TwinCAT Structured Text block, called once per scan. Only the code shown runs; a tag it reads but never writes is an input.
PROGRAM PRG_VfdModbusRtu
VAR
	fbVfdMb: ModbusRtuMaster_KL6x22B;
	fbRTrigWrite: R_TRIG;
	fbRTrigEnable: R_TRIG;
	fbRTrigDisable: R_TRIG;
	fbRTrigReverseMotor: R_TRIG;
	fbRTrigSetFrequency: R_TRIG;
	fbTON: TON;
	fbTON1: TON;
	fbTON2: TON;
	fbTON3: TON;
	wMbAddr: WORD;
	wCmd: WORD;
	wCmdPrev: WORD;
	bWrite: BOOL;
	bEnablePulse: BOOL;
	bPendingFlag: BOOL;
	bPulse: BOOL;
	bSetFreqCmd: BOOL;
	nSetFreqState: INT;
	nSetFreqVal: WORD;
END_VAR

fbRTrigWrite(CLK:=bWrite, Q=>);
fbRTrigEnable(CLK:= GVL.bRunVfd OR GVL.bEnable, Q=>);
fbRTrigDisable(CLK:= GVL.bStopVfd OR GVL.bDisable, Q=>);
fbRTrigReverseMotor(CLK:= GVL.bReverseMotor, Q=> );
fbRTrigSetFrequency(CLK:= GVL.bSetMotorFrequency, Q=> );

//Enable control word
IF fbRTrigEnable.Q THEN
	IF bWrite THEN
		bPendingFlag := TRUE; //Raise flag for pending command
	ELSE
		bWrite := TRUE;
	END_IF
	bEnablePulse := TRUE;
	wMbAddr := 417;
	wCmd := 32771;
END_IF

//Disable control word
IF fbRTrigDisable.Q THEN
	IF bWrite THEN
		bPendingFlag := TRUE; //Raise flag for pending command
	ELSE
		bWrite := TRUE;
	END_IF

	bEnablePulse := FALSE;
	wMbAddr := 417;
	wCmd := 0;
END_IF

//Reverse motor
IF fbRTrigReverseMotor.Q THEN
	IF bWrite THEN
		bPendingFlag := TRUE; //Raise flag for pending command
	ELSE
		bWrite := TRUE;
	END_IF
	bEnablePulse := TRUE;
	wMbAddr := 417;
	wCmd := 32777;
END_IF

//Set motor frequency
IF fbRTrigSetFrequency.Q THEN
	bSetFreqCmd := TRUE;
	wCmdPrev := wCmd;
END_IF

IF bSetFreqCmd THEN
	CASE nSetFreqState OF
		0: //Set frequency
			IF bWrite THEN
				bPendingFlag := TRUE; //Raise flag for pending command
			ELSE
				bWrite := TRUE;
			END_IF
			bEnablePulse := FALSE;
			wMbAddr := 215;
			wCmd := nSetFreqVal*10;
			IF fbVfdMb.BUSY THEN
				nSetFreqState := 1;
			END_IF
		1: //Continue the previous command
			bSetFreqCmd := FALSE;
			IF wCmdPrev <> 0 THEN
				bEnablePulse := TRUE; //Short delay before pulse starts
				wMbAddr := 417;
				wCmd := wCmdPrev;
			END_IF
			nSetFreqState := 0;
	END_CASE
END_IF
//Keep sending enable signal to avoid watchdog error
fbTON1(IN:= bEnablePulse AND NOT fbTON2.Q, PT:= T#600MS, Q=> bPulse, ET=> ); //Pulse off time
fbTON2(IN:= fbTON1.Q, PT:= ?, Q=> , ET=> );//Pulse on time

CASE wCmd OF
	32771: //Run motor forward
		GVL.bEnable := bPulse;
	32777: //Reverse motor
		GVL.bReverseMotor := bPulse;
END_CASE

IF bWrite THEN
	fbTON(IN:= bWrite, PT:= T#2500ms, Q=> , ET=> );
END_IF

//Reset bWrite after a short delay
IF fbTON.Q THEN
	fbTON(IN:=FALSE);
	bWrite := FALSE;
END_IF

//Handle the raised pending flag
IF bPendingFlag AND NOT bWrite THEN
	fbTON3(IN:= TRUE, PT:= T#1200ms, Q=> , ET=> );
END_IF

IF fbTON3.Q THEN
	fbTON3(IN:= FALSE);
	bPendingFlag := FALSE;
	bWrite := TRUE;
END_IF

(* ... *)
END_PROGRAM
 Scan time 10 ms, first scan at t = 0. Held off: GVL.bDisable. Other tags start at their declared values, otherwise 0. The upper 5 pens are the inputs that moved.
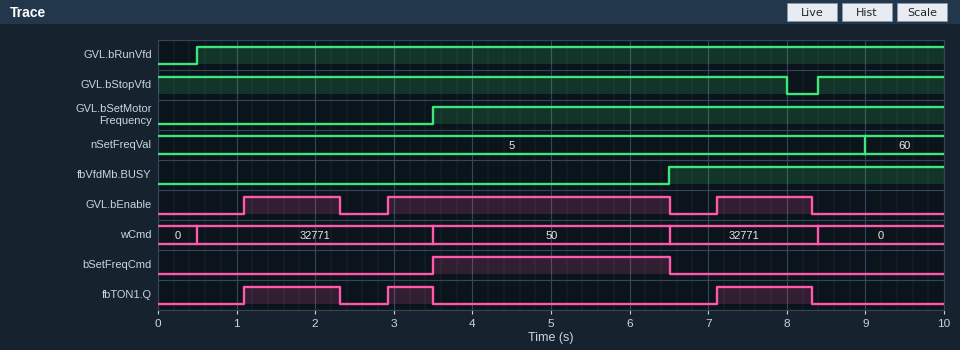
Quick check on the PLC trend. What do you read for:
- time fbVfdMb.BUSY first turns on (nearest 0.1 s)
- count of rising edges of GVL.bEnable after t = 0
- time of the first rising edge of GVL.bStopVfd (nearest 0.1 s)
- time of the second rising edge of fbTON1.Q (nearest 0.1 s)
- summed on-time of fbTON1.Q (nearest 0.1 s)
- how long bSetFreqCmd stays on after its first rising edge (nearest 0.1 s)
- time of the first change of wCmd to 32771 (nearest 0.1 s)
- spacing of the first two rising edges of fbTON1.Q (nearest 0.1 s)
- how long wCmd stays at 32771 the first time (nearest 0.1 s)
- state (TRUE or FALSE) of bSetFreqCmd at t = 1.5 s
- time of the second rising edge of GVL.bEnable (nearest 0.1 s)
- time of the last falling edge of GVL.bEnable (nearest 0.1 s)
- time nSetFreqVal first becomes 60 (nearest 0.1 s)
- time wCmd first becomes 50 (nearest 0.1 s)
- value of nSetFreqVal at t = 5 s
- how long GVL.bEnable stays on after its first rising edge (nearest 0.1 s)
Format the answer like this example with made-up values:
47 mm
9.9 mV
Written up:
6.5 s
3
8.4 s
2.9 s
3.0 s
3.0 s
0.5 s
1.8 s
3.0 s
FALSE
2.9 s
8.3 s
9.0 s
3.5 s
5
1.2 s
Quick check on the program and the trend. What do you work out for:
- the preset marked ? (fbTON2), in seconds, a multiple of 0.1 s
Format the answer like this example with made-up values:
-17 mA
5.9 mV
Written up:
1.2 s
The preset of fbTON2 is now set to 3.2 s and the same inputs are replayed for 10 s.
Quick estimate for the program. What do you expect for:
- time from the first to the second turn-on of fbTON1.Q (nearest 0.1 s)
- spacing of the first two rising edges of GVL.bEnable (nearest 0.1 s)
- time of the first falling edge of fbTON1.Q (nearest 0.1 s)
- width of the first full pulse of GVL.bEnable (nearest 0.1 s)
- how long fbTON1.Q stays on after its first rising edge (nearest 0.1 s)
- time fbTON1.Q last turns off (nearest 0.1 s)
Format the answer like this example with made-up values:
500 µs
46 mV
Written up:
6.0 s
6.0 s
3.5 s
5.4 s
2.4 s
8.4 s
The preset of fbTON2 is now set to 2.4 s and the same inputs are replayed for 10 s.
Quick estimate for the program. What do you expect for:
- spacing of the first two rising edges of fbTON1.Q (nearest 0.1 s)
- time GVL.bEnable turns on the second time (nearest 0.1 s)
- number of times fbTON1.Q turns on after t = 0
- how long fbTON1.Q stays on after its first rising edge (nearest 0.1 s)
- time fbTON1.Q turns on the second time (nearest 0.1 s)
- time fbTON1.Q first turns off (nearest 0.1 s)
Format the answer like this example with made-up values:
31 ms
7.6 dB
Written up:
6.0 s
7.1 s
2
2.4 s
7.1 s
3.5 s
